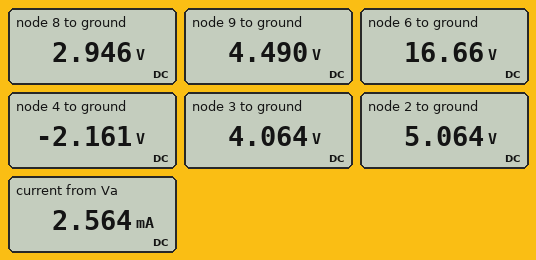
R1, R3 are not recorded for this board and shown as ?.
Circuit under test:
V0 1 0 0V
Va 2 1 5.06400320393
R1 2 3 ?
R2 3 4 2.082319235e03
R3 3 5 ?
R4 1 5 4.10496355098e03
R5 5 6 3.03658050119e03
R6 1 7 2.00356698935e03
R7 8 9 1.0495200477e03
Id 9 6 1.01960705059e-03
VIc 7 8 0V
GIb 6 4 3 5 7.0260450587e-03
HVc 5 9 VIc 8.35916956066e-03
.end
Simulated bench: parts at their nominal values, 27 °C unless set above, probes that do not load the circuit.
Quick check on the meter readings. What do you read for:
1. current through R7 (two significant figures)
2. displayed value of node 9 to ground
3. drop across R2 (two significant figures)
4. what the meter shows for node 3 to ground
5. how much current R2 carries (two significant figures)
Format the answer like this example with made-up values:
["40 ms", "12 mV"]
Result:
["1.5 mA", "4.490 V", "6.2 V", "4.064 V", "3.0 mA"]
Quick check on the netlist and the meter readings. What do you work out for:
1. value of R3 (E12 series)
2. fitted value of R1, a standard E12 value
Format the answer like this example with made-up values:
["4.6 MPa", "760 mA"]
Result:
["1 kΩ", "390 Ω"]
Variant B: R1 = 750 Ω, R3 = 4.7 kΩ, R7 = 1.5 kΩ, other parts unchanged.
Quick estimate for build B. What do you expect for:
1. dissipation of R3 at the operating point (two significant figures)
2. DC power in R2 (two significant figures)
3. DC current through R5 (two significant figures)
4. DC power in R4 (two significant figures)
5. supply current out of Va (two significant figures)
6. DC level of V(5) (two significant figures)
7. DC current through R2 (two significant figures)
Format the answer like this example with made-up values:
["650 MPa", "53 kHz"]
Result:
["19 µW", "9.1 mW", "3.1 mA", "3.6 mW", "2.0 mA", "3.8 V", "2.1 mA"]
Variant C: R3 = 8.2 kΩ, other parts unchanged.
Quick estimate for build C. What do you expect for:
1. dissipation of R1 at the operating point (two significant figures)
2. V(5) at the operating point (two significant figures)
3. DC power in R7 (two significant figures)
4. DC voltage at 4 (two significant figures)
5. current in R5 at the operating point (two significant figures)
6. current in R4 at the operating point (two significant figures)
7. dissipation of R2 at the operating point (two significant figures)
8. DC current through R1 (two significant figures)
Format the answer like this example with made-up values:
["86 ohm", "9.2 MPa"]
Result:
["2.5 mW", "4.4 V", "2.2 mW", "-1.3 V", "3.6 mA", "1.1 mA", "14 mW", "2.5 mA"]
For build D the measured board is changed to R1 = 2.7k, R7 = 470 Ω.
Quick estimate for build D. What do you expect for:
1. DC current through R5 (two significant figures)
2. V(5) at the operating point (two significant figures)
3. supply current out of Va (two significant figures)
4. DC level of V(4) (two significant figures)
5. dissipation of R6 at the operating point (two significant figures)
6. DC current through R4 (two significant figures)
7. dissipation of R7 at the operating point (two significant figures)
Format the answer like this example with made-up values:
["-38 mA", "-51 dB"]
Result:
["2.5 mA", "1.9 V", "1.2 mA", "-1.3 V", "1.2 mW", "470 µA", "280 µW"]
